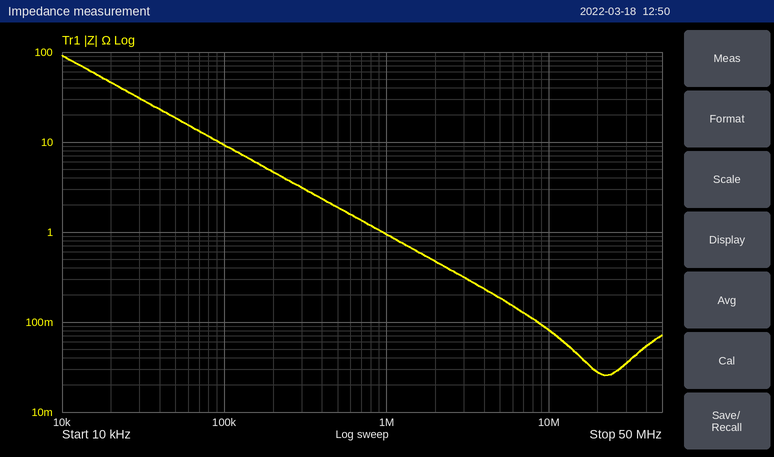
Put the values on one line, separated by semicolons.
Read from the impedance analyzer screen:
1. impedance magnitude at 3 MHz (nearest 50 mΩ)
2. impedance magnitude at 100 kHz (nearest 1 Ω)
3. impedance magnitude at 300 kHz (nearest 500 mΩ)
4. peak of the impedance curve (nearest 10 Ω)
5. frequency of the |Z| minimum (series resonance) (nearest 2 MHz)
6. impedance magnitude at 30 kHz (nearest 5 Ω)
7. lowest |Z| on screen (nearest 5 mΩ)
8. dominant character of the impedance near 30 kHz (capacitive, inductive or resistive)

300 mΩ; 9 Ω; 3.0 Ω; 90 Ω; 22 MHz; 30 Ω; 25 mΩ; capacitive
